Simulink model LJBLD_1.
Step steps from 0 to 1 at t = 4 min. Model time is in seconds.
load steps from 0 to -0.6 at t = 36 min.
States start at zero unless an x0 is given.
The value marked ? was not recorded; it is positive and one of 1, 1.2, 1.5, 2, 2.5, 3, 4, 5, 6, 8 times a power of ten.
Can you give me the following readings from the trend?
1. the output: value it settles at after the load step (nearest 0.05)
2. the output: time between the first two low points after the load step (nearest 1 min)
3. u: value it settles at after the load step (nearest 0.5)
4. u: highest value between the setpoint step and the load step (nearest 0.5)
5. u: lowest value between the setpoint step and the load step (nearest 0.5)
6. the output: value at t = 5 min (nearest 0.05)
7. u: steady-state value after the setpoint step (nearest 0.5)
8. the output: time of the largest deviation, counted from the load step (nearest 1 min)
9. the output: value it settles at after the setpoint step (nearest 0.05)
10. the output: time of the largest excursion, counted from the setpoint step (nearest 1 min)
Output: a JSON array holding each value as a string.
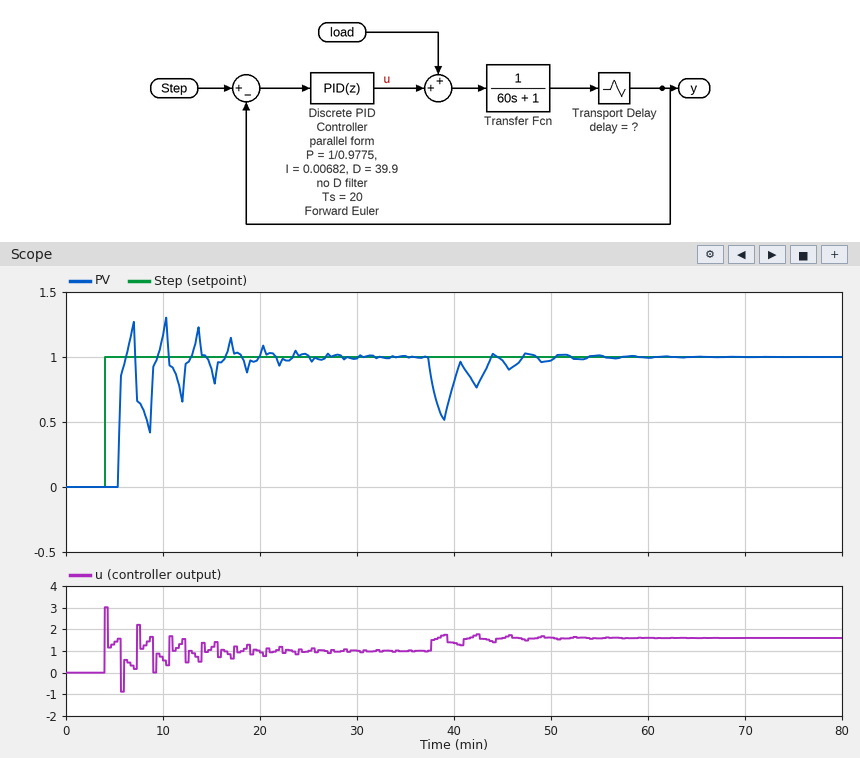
["1.00", "3 min", "1.5", "3.0", "-1.0", "0.00", "1.0", "3 min", "1.00", "6 min"]
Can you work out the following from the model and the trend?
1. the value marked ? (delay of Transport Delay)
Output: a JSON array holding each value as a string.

["80"]
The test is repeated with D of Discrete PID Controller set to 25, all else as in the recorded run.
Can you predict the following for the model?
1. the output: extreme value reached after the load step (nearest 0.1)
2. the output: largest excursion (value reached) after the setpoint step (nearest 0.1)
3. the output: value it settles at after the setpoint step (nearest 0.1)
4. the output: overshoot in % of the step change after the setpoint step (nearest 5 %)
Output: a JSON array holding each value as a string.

["0.5", "1.2", "1.0", "20 %"]
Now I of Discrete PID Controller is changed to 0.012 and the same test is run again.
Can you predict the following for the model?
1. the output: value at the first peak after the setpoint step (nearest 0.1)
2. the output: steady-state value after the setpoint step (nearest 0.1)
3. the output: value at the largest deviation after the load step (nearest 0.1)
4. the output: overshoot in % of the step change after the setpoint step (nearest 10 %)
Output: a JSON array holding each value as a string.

["1.5", "1.0", "0.5", "50 %"]
